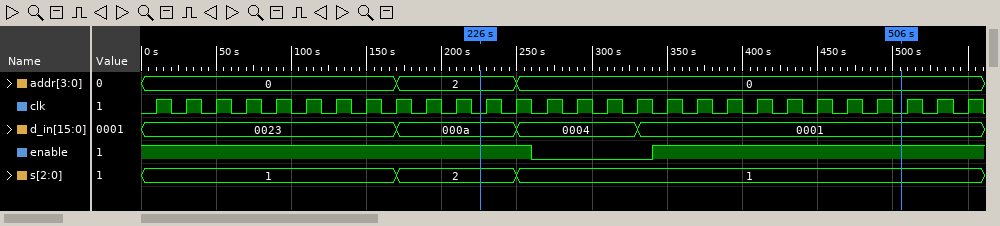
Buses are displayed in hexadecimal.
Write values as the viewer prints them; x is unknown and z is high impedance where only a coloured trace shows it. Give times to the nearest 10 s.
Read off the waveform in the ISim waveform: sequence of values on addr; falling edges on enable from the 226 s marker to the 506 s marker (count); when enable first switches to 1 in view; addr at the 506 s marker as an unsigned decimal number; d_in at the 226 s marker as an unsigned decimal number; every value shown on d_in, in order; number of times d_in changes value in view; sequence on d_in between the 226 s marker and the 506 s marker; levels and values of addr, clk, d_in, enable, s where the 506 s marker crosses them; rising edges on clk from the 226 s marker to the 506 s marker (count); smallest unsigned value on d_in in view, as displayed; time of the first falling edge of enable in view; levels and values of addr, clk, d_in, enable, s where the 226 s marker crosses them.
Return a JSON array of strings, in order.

["0, 2, 0", "1", "340 s", "0", "10", "0023, 000a, 0004, 0001", "3", "000a, 0004, 0001", "addr=0, clk=0, d_in=0001, enable=1, s=1", "14", "0001", "260 s", "addr=2, clk=0, d_in=000a, enable=1, s=2"]
